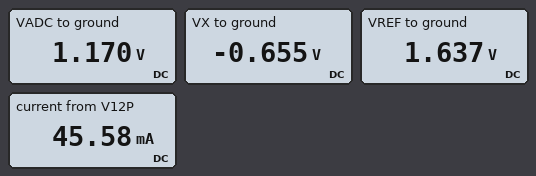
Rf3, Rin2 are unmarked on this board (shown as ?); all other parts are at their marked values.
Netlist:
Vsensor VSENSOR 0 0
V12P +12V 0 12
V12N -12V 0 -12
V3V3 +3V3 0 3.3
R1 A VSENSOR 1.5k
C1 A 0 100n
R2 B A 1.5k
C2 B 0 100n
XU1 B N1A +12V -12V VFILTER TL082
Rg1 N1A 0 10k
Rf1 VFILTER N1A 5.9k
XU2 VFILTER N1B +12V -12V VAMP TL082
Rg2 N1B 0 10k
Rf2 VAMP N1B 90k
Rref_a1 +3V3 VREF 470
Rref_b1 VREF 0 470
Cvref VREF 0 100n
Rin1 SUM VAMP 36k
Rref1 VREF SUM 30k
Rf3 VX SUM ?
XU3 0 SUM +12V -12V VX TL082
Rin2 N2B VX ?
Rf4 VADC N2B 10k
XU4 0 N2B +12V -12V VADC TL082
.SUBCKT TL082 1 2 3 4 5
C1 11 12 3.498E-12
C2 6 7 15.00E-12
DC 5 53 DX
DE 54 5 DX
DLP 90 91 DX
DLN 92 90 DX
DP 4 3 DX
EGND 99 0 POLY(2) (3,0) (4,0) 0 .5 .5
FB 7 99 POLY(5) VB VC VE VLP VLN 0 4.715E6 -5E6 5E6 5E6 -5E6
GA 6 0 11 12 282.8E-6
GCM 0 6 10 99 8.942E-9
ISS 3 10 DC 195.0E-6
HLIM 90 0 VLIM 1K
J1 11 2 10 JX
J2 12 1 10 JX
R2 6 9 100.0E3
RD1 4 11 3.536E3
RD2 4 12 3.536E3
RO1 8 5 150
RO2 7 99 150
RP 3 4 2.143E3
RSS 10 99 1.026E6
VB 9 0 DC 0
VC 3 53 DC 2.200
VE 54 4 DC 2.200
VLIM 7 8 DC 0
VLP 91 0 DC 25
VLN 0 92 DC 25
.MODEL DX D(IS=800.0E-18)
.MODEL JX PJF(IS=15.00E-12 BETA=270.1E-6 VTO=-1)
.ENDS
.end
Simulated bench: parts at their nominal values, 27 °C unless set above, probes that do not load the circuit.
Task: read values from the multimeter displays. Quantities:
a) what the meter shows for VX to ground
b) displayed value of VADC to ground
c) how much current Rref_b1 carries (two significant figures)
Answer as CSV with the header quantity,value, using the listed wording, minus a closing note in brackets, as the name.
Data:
quantity,value
what the meter shows for VX to ground,-0.655 V
displayed value of VADC to ground,1.170 V
how much current Rref_b1 carries,3.5 mA
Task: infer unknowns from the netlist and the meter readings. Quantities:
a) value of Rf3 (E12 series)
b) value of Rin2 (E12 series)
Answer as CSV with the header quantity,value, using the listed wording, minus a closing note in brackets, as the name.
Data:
quantity,value
value of Rf3,12 kΩ
value of Rin2,5.6 kΩ
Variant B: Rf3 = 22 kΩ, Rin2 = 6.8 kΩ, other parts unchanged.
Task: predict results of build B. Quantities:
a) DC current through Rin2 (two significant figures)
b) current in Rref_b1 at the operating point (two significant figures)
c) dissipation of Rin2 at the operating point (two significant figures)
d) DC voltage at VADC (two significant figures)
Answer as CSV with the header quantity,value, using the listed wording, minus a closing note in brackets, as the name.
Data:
quantity,value
DC current through Rin2,180 µA
current in Rref_b1 at the operating point,3.5 mA
dissipation of Rin2 at the operating point,210 µW
DC voltage at VADC,1.8 V
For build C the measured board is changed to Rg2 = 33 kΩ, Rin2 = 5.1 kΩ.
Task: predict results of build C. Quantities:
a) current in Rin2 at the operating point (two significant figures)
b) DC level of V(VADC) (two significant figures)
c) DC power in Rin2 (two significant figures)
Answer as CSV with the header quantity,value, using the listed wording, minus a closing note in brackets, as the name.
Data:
quantity,value
current in Rin2 at the operating point,130 µA
DC level of V(VADC),1.3 V
DC power in Rin2,84 µW
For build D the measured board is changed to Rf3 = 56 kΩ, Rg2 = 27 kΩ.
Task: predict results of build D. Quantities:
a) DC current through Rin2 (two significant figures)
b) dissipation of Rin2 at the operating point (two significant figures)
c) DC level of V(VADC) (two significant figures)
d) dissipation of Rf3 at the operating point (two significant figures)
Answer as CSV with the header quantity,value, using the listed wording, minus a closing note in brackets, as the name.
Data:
quantity,value
DC current through Rin2,550 µA
dissipation of Rin2 at the operating point,1.7 mW
DC level of V(VADC),5.5 V
dissipation of Rf3 at the operating point,170 µW
